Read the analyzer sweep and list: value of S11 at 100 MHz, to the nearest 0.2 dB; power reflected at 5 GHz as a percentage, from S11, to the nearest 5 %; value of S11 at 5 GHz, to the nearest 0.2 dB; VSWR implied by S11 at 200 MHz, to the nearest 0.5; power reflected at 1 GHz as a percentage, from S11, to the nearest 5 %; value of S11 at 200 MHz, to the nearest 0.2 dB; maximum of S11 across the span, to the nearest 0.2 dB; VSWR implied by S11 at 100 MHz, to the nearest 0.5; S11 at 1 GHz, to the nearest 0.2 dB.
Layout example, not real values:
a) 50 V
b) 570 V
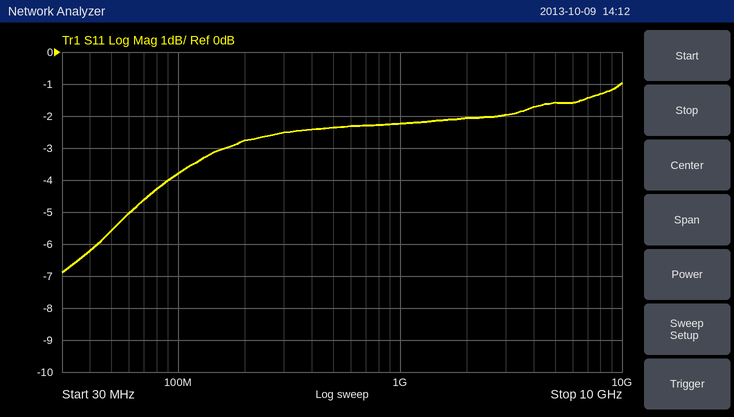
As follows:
a) -3.8 dB
b) 70 %
c) -1.6 dB
d) 6.5
e) 60 %
f) -2.8 dB
g) -1.0 dB
h) 4.5
i) -2.2 dB
